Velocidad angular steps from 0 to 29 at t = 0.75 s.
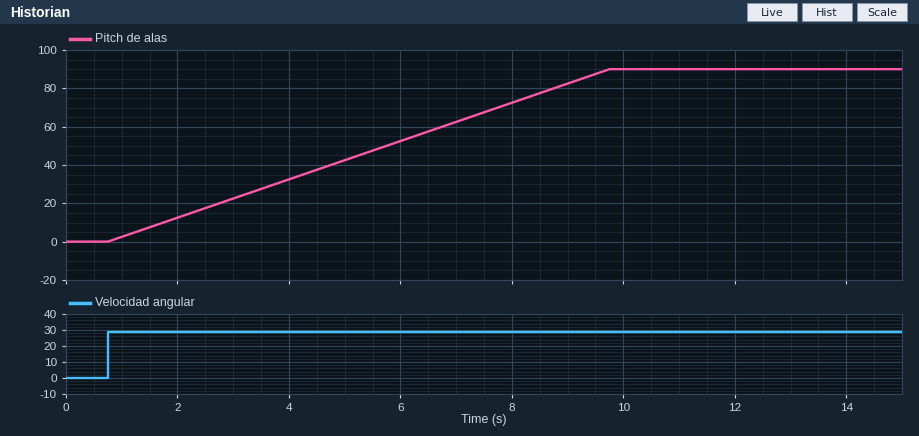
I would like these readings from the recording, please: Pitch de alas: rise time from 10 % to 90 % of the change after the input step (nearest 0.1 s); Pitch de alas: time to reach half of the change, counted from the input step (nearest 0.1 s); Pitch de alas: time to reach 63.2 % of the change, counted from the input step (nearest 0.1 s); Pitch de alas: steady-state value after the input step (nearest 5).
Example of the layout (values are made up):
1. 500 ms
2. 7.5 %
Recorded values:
1. 7.2 s
2. 4.5 s
3. 5.7 s
4. 90
